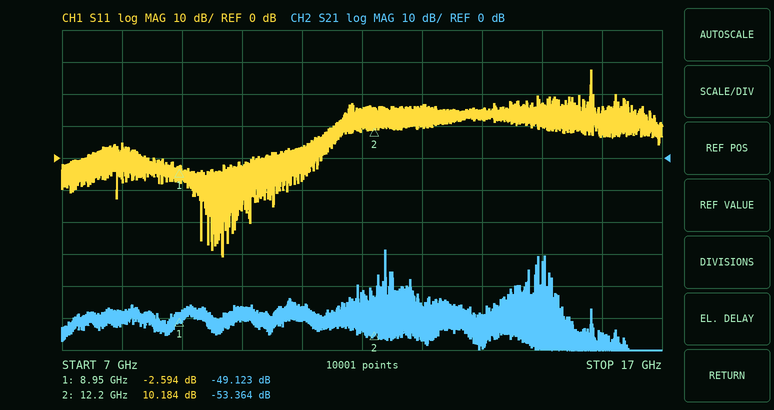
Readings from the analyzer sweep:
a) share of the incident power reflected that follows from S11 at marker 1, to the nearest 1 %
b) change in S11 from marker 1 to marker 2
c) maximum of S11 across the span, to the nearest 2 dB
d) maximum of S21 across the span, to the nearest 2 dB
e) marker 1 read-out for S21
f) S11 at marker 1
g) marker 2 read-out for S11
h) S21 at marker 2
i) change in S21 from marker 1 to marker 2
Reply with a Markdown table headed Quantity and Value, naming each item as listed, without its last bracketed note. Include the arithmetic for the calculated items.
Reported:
| Quantity | Value |
|---|---|
| share of the incident power reflected that follows from S11 at marker 1, to the nearest 1 % | 10^(-2.594/10) ≈ 55 % |
| change in S11 from marker 1 to marker 2 | 10.184 − (-2.594) = 12.778 dB |
| maximum of S11 across the span, to the nearest 2 dB | 28 dB |
| maximum of S21 across the span, to the nearest 2 dB | -28 dB |
| marker 1 read-out for S21 | -49.123 dB |
| S11 at marker 1 | -2.594 dB |
| marker 2 read-out for S11 | 10.184 dB |
| S21 at marker 2 | -53.364 dB |
| change in S21 from marker 1 to marker 2 | -53.364 − (-49.123) = -4.241 dB |
